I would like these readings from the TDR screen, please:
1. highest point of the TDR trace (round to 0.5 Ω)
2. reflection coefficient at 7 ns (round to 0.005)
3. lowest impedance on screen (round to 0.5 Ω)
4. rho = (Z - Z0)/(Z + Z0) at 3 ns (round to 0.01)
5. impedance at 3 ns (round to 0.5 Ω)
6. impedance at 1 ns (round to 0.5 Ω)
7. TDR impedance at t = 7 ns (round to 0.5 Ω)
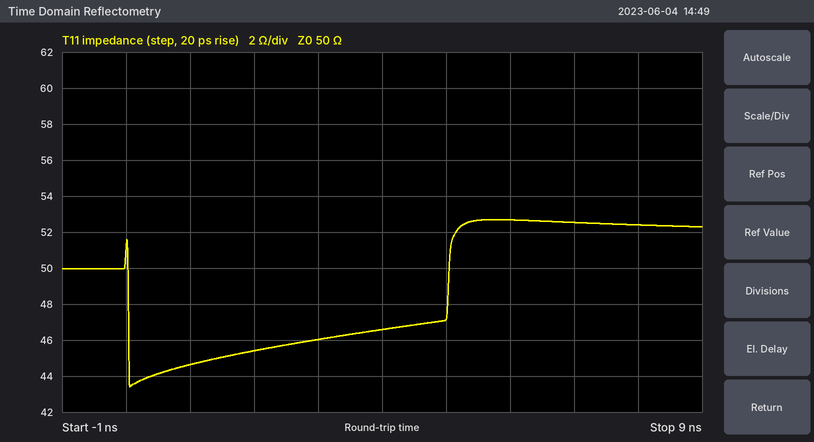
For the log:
52.5 Ω
+0.025
43.5 Ω
-0.04
46.0 Ω
44.5 Ω
52.5 Ω
